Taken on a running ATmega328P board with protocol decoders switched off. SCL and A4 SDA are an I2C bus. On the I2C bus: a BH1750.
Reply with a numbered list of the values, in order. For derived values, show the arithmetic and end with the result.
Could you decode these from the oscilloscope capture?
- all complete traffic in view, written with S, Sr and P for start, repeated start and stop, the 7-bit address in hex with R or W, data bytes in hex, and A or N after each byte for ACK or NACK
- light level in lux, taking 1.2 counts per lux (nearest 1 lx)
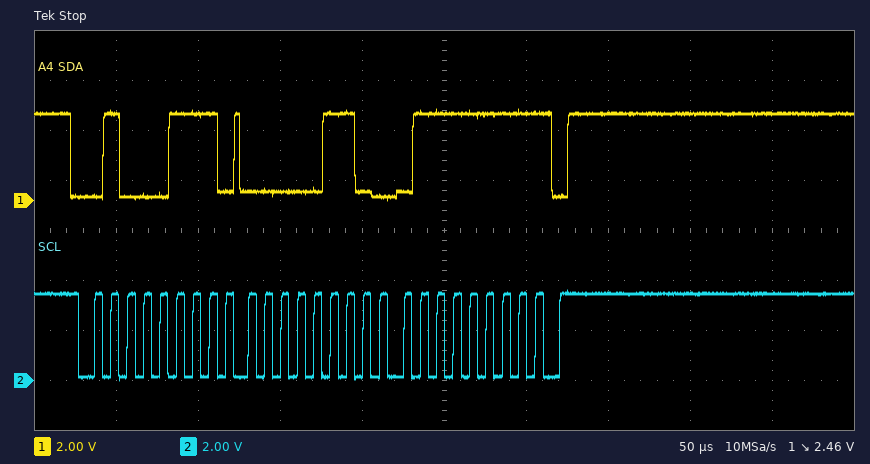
1. S 23R A 06 A 7F N P
2. 1663 / 1.2 = 1386 lx
